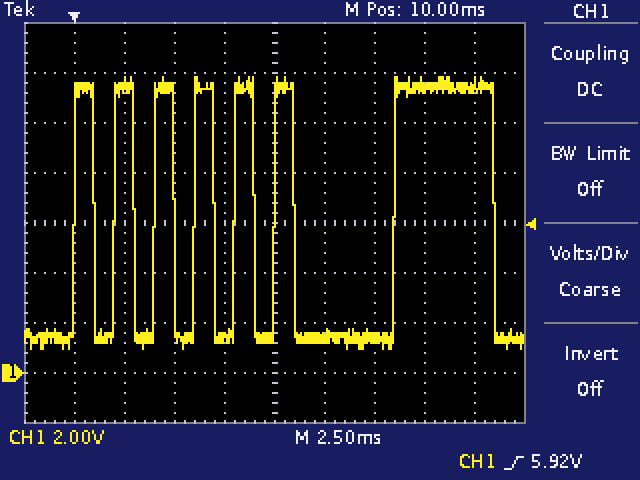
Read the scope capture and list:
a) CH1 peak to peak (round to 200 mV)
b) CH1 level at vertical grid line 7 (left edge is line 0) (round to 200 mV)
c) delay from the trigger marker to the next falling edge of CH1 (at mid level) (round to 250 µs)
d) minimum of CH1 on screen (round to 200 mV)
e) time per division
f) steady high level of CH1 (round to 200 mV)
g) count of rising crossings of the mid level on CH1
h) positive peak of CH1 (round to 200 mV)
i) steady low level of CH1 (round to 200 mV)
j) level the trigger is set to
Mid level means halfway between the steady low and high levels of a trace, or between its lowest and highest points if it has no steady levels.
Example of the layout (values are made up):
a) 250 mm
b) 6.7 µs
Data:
a) 10.8 V
b) 1.4 V
c) 1.00 ms
d) 1.0 V
e) 2.5 ms
f) 11.4 V
g) 7
h) 11.8 V
i) 1.4 V
j) 5.92 V
